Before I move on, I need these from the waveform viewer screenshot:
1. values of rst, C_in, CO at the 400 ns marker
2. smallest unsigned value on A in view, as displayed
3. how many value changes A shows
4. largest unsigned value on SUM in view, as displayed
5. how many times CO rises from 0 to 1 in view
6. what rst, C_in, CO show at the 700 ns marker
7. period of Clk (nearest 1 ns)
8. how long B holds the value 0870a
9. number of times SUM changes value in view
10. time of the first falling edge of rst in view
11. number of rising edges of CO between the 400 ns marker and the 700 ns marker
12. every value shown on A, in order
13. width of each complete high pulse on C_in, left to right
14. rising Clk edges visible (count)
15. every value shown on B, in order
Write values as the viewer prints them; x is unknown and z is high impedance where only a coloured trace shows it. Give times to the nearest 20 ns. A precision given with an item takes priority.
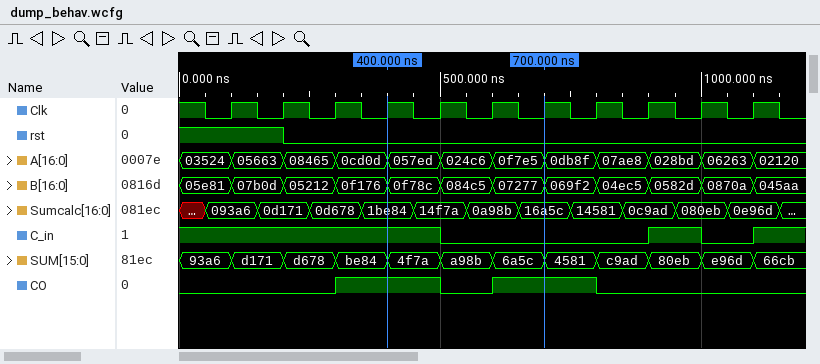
rst=0, C_in=1, CO=1
02120
11
e96d
2
rst=0, C_in=0, CO=1
100 ns
100 ns
11
200 ns
1
03524, 05663, 08465, 0cd0d, 057ed, 024c6, 0f7e5, 0db8f, 07ae8, 028bd, 06263, 02120
100 ns
11
05e81, 07b0d, 05212, 0f176, 0f78c, 084c5, 07277, 069f2, 04ec5, 0582d, 0870a, 045aa
